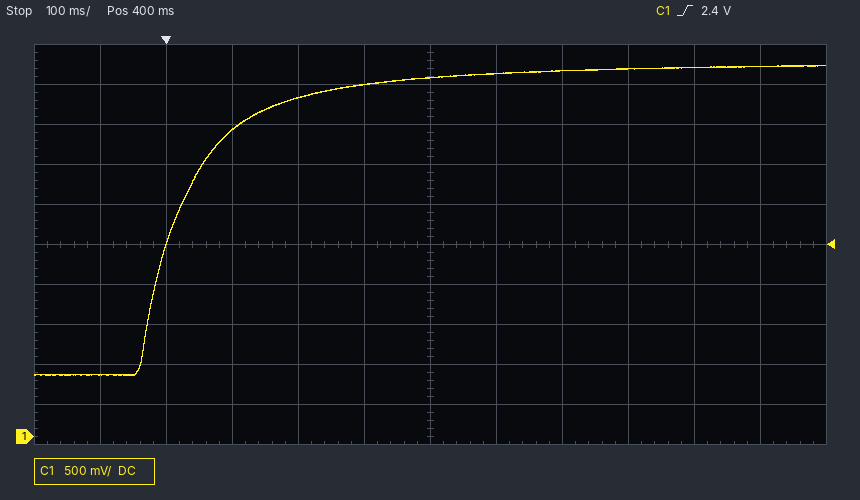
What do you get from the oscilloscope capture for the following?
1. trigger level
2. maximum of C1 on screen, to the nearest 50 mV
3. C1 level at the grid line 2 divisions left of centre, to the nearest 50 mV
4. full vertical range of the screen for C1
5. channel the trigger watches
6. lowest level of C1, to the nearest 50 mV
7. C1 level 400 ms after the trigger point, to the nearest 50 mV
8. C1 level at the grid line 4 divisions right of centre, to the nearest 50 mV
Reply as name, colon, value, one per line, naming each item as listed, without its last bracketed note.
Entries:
trigger level: 2.4 V
maximum of C1 on screen, to the nearest 50 mV: 4.65 V
C1 level at the grid line 2 divisions left of centre, to the nearest 50 mV: 4.25 V
full vertical range of the screen for C1: 5 V
channel the trigger watches: C1
lowest level of C1, to the nearest 50 mV: 750 mV
C1 level 400 ms after the trigger point, to the nearest 50 mV: 4.50 V
C1 level at the grid line 4 divisions right of centre, to the nearest 50 mV: 4.60 V
